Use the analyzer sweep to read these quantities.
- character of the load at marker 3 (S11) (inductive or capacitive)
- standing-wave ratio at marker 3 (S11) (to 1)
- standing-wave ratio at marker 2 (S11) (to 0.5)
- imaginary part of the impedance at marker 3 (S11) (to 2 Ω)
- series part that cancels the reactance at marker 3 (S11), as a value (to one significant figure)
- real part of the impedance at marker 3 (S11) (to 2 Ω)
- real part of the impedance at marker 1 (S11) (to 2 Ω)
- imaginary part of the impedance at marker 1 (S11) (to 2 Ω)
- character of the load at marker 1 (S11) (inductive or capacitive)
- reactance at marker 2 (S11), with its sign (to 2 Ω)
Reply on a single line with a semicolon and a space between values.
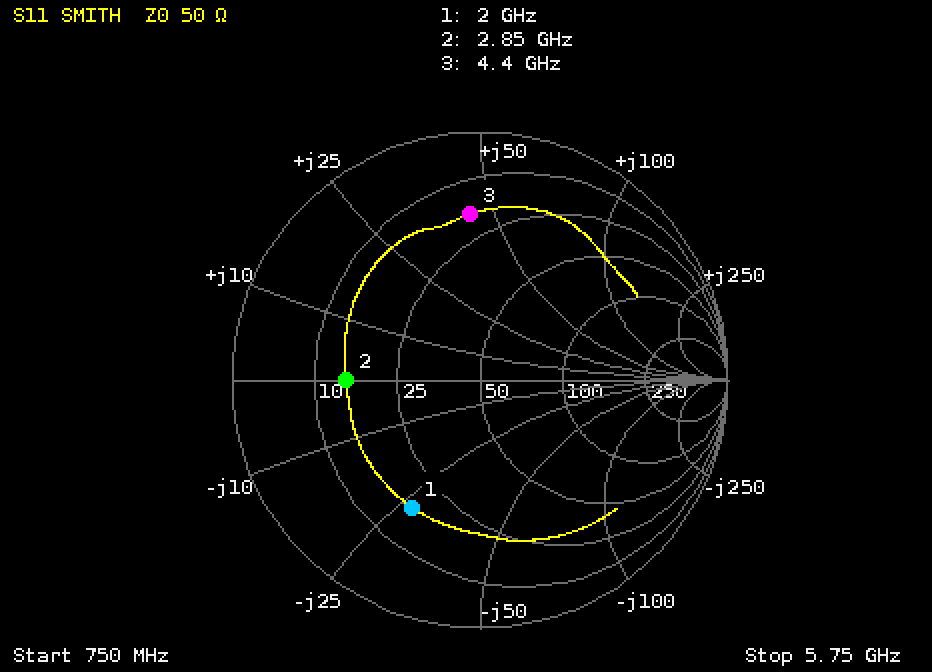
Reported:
inductive; 5; 3.5; +44 Ω; 800 fF; 18 Ω; 18 Ω; -28 Ω; capacitive; 0 Ω
